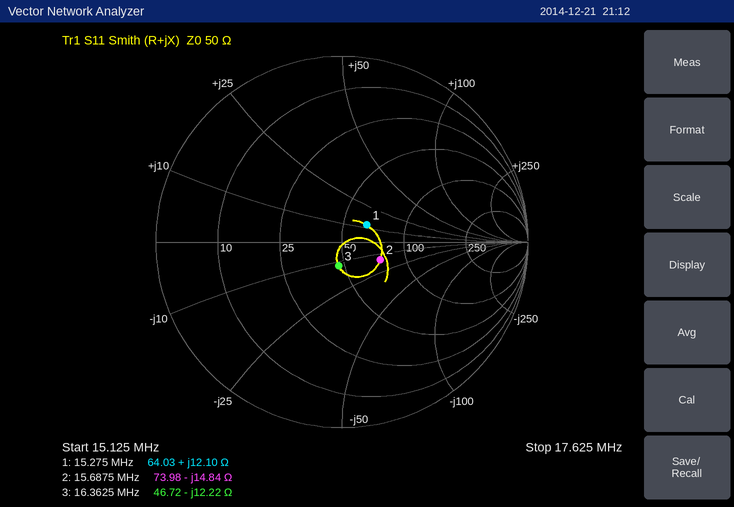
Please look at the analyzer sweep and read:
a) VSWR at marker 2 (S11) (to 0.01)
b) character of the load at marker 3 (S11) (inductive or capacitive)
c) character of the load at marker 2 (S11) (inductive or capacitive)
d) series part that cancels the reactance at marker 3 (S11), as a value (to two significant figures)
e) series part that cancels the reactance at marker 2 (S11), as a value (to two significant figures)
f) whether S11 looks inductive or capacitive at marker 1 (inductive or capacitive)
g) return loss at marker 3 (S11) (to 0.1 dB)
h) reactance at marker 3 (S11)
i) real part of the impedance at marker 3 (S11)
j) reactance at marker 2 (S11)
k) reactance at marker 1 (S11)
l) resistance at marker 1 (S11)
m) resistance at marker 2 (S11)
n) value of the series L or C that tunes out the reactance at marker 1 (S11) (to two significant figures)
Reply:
1.58
capacitive
capacitive
120 nH
150 nH
inductive
17.7 dB
-12.22 Ω
46.72 Ω
-14.84 Ω
+12.10 Ω
64.03 Ω
73.98 Ω
860 pF
